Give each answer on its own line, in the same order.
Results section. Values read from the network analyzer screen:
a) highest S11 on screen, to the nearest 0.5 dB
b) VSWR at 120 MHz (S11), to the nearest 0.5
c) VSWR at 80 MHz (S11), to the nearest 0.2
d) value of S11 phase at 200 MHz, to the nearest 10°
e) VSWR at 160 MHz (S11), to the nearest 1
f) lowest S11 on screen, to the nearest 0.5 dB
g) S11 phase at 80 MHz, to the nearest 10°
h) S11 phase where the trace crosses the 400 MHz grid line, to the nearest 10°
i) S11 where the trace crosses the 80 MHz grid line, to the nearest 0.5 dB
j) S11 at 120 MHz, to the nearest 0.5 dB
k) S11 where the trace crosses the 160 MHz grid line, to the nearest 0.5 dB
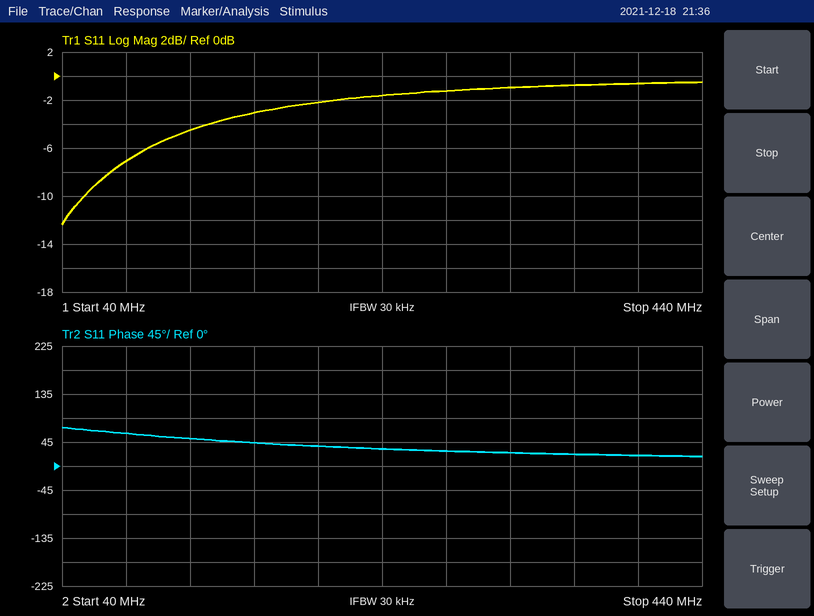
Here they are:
-0.5 dB
4.0
2.6
40°
6
-12.5 dB
60°
20°
-7.0 dB
-4.5 dB
-3.0 dB
